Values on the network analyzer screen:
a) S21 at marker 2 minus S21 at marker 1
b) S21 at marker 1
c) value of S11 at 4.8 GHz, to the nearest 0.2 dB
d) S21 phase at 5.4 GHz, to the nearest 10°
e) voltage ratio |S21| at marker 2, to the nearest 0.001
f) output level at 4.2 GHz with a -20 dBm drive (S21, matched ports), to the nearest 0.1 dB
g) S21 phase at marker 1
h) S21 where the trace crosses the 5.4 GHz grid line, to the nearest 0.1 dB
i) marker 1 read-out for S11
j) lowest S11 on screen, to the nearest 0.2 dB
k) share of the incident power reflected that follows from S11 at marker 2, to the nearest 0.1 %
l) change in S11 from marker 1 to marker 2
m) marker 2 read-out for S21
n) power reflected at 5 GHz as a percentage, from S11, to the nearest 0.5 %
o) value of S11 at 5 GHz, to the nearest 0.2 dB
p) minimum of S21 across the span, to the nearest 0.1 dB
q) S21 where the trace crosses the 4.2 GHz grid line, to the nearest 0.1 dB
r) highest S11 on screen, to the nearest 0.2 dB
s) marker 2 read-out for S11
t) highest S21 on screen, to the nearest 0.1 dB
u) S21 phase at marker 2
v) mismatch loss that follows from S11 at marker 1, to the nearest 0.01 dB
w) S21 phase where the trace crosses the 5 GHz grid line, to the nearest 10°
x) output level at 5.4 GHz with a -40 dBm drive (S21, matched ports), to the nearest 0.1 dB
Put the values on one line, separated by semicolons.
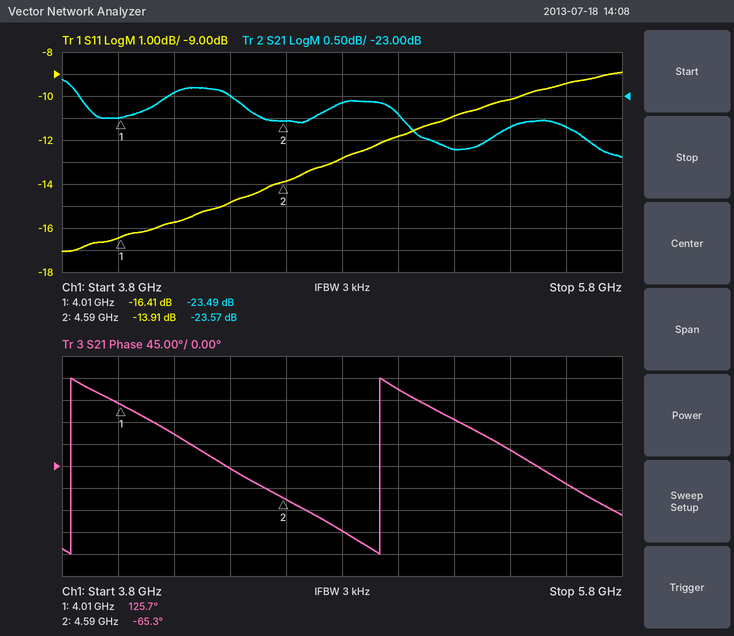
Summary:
-0.08 dB; -23.49 dB; -12.8 dB; 30°; 0.066; -42.9 dBm; 125.7°; -23.7 dB; -16.41 dB; -17.0 dB; 4.1 %; 2.50 dB; -23.57 dB; 6.5 %; -11.8 dB; -24.4 dB; -22.9 dB; -9.0 dB; -13.91 dB; -22.6 dB; -65.3°; 0.10 dB; 160°; -63.7 dBm
